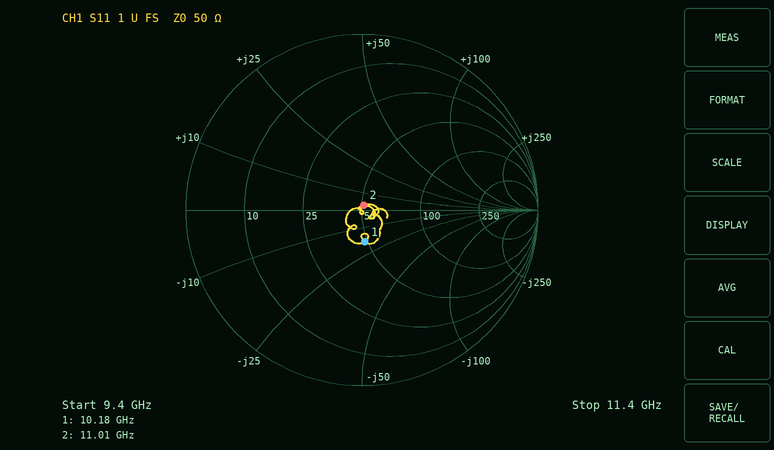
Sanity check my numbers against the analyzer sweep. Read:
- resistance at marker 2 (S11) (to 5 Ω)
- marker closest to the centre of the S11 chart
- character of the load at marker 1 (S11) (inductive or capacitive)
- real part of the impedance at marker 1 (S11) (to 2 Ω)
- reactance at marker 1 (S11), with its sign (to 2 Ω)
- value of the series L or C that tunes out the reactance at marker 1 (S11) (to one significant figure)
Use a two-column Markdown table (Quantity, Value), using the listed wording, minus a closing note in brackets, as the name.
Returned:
| Quantity | Value |
|---|---|
| resistance at marker 2 (S11) | 50 Ω |
| marker closest to the centre of the S11 chart | marker 2 |
| character of the load at marker 1 (S11) | capacitive |
| real part of the impedance at marker 1 (S11) | 48 Ω |
| reactance at marker 1 (S11), with its sign | -18 Ω |
| value of the series L or C that tunes out the reactance at marker 1 (S11) | 300 pH |
